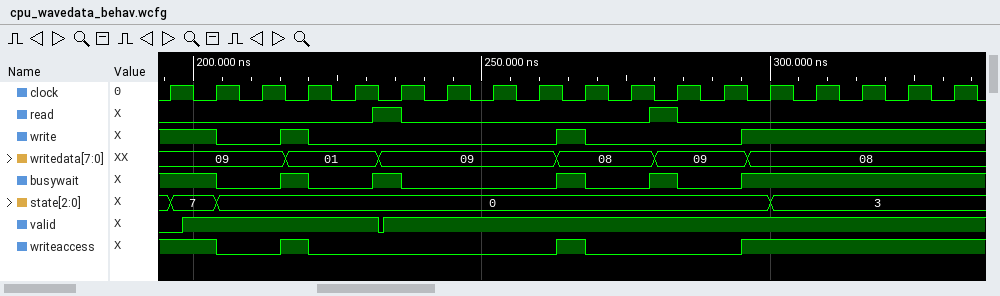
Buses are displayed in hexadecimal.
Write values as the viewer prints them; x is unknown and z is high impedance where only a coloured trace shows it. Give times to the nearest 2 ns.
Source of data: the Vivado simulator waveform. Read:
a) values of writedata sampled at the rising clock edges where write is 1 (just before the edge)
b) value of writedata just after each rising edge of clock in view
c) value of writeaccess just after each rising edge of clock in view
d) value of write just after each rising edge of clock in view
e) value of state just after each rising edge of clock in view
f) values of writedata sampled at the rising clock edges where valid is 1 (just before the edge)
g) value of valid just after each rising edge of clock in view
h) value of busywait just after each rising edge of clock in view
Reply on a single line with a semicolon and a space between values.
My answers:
09, 09, 01, 08, 08, 08, 08, 08, 08; 09, 09, 09, 01, 01, 09, 09, 09, 09, 08, 08, 09, 09, 08, 08, 08, 08, 08; 1 0 0 0 0 0 0 0 0 0 0 0 0 1 1 1 1 1; 1 0 0 0 0 0 0 0 0 0 0 0 0 1 1 1 1 1; 7, 0, 0, 0, 0, 0, 0, 0, 0, 0, 0, 0, 0, 3, 3, 3, 3, 3; 09, 09, 01, 01, 09, 09, 09, 09, 08, 08, 09, 09, 08, 08, 08, 08, 08; 0 1 1 1 1 1 1 1 1 1 1 1 1 1 1 1 1 1; 1 0 0 0 0 0 0 0 0 0 0 0 0 1 1 1 1 1
